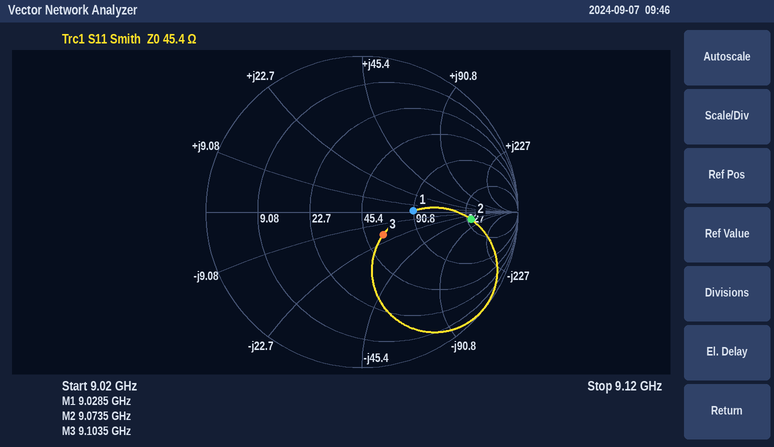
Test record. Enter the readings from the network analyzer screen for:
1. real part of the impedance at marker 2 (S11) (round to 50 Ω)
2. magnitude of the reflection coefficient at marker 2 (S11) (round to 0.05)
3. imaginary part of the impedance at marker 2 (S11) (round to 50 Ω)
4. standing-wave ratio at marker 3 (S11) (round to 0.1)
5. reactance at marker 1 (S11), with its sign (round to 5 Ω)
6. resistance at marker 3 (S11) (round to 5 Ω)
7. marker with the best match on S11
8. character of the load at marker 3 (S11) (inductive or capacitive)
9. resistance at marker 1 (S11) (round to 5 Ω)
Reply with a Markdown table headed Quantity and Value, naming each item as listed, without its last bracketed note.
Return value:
| Quantity | Value |
|---|---|
| real part of the impedance at marker 2 (S11) | 250 Ω |
| magnitude of the reflection coefficient at marker 2 (S11) | 0.70 |
| imaginary part of the impedance at marker 2 (S11) | -50 Ω |
| standing-wave ratio at marker 3 (S11) | 1.5 |
| reactance at marker 1 (S11), with its sign | 0 Ω |
| resistance at marker 3 (S11) | 55 Ω |
| marker with the best match on S11 | marker 3 |
| character of the load at marker 3 (S11) | capacitive |
| resistance at marker 1 (S11) | 90 Ω |
